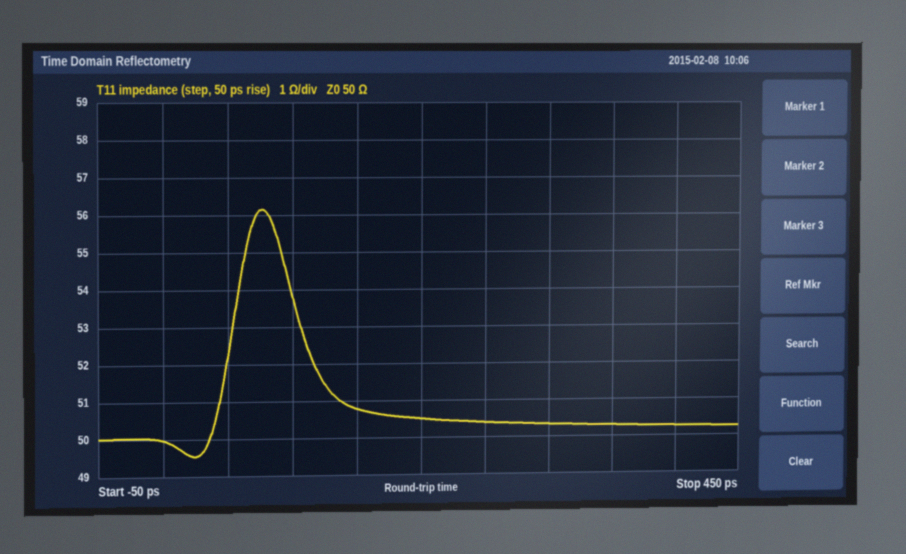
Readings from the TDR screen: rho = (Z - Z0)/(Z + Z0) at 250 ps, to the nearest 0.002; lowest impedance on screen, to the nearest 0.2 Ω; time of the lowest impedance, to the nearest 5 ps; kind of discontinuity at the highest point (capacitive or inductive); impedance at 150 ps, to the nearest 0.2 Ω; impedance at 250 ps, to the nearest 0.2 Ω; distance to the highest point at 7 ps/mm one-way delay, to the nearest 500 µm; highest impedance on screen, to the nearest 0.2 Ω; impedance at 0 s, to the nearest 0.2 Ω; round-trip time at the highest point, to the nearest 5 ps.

+0.004
49.6 Ω
25 ps
inductive
50.8 Ω
50.4 Ω
5.5 mm
56.2 Ω
50.0 Ω
75 ps
